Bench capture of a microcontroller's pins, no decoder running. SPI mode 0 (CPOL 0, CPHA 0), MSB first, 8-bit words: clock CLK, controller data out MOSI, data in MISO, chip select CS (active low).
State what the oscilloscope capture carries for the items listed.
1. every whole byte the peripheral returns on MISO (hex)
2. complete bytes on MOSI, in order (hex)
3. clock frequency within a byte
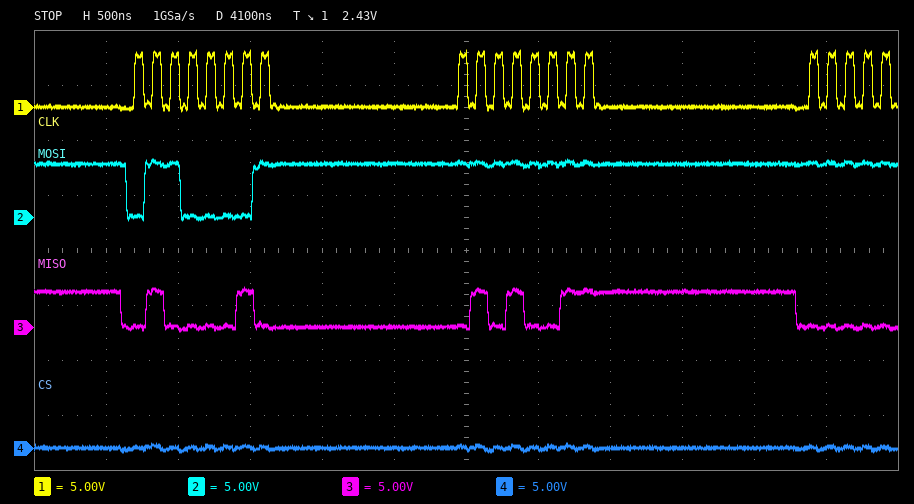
42 53
61 FF
8 MHz
